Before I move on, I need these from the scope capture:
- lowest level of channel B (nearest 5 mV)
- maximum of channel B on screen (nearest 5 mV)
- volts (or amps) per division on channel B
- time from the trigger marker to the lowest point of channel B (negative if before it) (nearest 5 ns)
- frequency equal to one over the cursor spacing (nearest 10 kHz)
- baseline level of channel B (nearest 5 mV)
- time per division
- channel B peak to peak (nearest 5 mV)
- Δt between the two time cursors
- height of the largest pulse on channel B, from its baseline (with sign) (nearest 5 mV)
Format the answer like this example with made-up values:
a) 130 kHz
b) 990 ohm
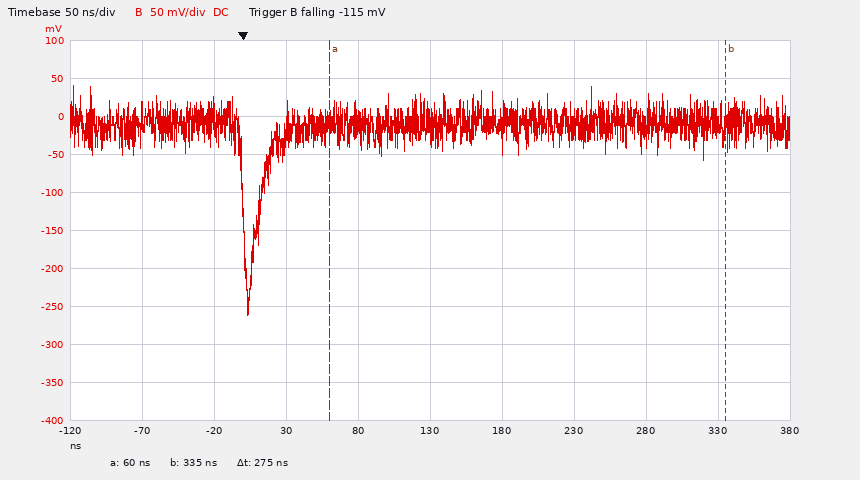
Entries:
a) -260 mV
b) 40 mV
c) 50 mV
d) +5 ns
e) 3.64 MHz
f) -10 mV
g) 50 ns
h) 300 mV
i) 275 ns
j) -250 mV
